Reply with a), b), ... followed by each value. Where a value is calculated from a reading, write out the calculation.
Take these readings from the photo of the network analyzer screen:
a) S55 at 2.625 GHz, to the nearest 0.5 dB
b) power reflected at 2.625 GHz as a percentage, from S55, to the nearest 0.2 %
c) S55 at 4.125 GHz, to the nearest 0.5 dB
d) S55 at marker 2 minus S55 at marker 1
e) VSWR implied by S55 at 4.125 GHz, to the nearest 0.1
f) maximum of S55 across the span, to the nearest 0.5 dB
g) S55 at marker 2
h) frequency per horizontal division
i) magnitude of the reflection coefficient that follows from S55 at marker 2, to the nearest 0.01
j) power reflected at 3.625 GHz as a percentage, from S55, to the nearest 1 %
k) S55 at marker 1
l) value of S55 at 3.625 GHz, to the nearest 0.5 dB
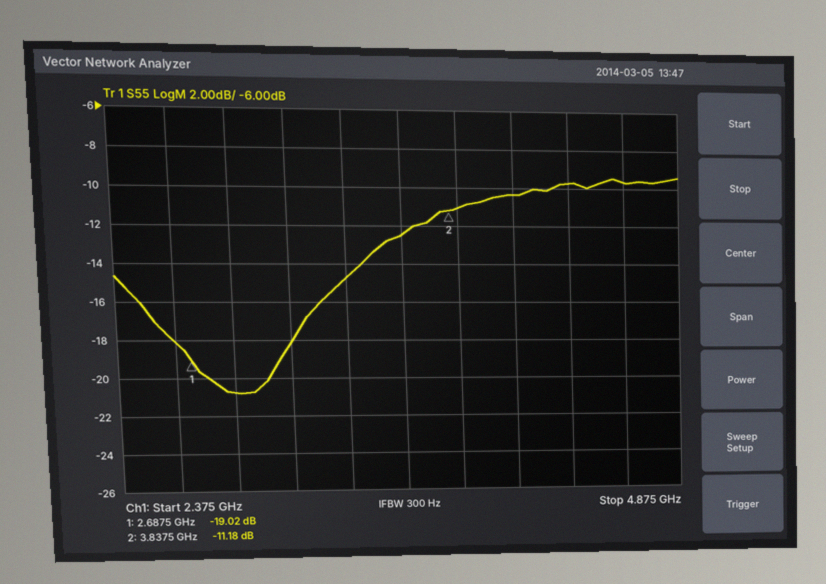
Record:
a) -18.0 dB
b) 10^(-18/10) ≈ 1.6 %
c) -10.5 dB
d) -11.18 − (-19.02) = 7.84 dB
e) |Γ| = 10^(-10.5/20) = 0.2985; VSWR = (1 + 0.2985)/(1 − 0.2985) ≈ 1.9
f) -9.5 dB
g) -11.18 dB
h) 250 MHz
i) 10^(-11.18/20) ≈ 0.28
j) 10^(-12.5/10) ≈ 6 %
k) -19.02 dB
l) -12.5 dB
